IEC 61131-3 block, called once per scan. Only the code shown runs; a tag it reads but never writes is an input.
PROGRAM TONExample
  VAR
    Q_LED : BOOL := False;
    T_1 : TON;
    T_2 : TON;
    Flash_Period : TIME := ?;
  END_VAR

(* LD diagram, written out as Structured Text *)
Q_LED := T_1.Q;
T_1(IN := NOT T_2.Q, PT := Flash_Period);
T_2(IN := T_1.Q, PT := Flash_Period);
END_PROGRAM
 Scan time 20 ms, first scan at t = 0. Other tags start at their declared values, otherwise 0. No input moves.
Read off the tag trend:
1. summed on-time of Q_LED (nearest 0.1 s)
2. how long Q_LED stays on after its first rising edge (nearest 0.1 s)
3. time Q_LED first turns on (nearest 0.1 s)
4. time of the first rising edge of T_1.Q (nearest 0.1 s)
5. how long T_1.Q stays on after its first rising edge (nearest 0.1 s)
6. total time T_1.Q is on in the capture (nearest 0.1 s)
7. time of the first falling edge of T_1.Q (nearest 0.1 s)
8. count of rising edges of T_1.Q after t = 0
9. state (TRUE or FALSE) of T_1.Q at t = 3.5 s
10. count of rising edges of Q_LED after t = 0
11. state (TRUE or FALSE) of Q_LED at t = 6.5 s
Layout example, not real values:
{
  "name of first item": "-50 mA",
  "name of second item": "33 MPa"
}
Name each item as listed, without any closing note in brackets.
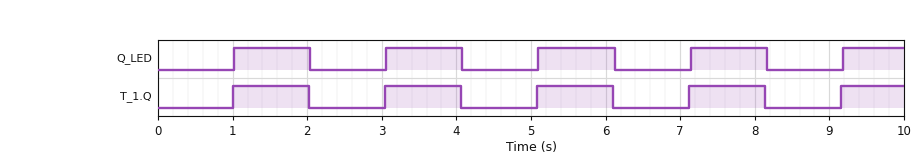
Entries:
{
  "summed on-time of Q_LED": "4.9 s",
  "how long Q_LED stays on after its first rising edge": "1.0 s",
  "time Q_LED first turns on": "1.0 s",
  "time of the first rising edge of T_1.Q": "1.0 s",
  "how long T_1.Q stays on after its first rising edge": "1.0 s",
  "total time T_1.Q is on in the capture": "4.9 s",
  "time of the first falling edge of T_1.Q": "2.0 s",
  "count of rising edges of T_1.Q after t = 0": "5",
  "state (TRUE or FALSE) of T_1.Q at t = 3.5 s": "TRUE",
  "count of rising edges of Q_LED after t = 0": "5",
  "state (TRUE or FALSE) of Q_LED at t = 6.5 s": "FALSE"
}
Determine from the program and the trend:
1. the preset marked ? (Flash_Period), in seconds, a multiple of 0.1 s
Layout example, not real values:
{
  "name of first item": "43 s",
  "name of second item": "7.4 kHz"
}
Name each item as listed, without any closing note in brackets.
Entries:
{
  "the preset marked ? (Flash_Period), in seconds, a multiple of 0.1 s": "1.0 s"
}
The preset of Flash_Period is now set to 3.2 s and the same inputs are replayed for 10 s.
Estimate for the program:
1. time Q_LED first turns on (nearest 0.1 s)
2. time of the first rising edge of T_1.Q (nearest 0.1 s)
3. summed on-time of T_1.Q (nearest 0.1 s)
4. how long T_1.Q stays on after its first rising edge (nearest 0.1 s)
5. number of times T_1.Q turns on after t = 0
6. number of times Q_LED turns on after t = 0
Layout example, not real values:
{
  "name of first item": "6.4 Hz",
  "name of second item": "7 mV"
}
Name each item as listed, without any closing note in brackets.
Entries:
{
  "time Q_LED first turns on": "3.2 s",
  "time of the first rising edge of T_1.Q": "3.2 s",
  "summed on-time of T_1.Q": "3.6 s",
  "how long T_1.Q stays on after its first rising edge": "3.2 s",
  "number of times T_1.Q turns on after t = 0": "2",
  "number of times Q_LED turns on after t = 0": "2"
}
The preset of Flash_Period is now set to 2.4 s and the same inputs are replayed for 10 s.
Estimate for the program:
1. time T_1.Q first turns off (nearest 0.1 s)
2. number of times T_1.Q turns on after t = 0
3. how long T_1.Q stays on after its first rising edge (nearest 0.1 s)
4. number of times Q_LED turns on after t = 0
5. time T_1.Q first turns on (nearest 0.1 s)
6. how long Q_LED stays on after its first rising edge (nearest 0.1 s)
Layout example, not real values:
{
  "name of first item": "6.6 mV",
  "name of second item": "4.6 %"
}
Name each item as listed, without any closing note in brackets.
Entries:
{
  "time T_1.Q first turns off": "4.8 s",
  "number of times T_1.Q turns on after t = 0": "2",
  "how long T_1.Q stays on after its first rising edge": "2.4 s",
  "number of times Q_LED turns on after t = 0": "2",
  "time T_1.Q first turns on": "2.4 s",
  "how long Q_LED stays on after its first rising edge": "2.4 s"
}
